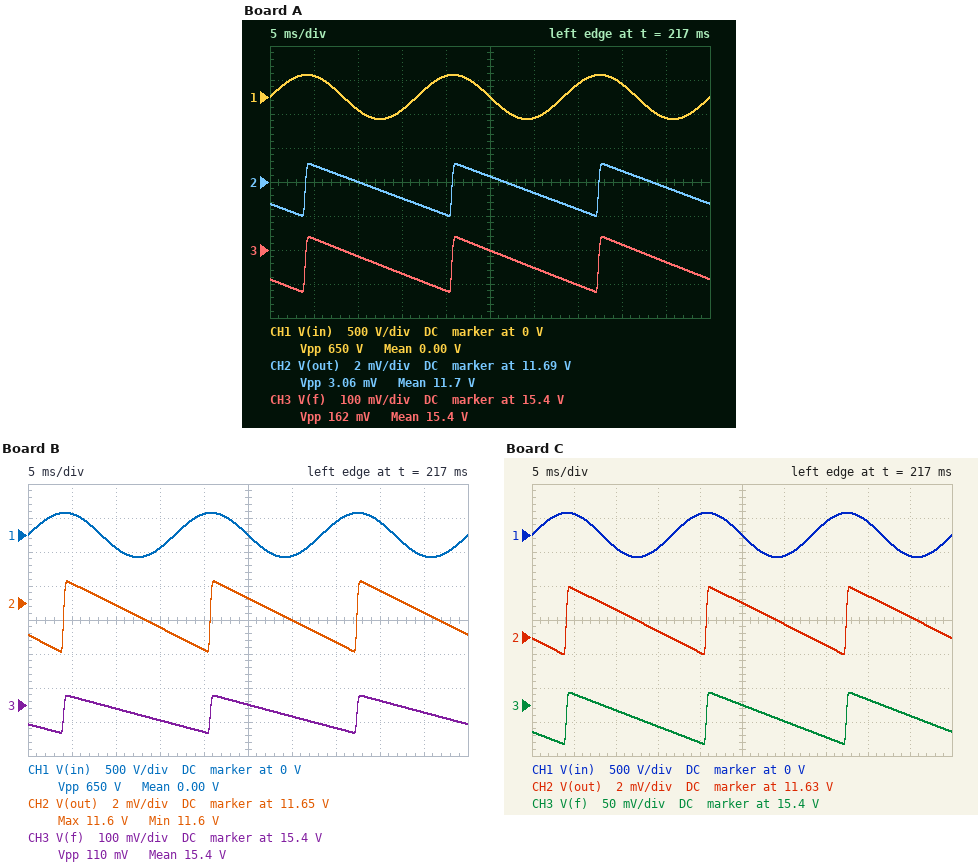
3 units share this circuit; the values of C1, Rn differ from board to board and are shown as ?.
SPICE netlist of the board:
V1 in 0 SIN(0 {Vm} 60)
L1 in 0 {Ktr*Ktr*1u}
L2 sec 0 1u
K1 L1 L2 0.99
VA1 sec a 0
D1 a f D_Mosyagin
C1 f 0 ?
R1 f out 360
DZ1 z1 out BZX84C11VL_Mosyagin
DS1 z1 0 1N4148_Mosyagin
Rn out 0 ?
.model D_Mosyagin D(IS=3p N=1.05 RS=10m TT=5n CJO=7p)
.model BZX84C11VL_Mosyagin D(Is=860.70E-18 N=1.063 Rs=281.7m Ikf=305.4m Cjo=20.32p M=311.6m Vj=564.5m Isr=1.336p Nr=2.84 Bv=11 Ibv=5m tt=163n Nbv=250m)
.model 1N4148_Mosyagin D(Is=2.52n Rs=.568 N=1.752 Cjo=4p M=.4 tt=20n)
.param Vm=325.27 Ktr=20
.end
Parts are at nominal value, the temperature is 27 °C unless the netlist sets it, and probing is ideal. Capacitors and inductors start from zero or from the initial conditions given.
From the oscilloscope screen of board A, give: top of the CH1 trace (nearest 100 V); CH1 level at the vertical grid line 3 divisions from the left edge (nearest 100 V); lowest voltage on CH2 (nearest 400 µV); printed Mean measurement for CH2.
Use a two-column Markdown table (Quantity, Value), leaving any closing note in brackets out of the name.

| Quantity | Value |
|---|---|
| top of the CH1 trace | 300 V |
| CH1 level at the vertical grid line 3 divisions from the left edge | -200 V |
| lowest voltage on CH2 | 11.6900 V |
| printed Mean measurement for CH2 | 11.7 V |
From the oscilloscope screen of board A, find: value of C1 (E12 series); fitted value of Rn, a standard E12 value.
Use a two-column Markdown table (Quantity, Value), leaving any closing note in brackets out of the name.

| Quantity | Value |
|---|---|
| value of C1 | 1 mF |
| fitted value of Rn, a standard E12 value | 6.8 kΩ |
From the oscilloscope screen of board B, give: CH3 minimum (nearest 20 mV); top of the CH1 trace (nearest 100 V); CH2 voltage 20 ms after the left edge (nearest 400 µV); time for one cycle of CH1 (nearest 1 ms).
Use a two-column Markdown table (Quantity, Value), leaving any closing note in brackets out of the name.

| Quantity | Value |
|---|---|
| CH3 minimum | 15.32 V |
| top of the CH1 trace | 300 V |
| CH2 voltage 20 ms after the left edge | 11.6452 V |
| time for one cycle of CH1 | 17 ms |
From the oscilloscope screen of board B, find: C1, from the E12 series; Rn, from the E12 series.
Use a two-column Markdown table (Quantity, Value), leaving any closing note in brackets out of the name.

| Quantity | Value |
|---|---|
| C1, from the E12 series | 1.5 mF |
| Rn, from the E12 series | 1.8 kΩ |
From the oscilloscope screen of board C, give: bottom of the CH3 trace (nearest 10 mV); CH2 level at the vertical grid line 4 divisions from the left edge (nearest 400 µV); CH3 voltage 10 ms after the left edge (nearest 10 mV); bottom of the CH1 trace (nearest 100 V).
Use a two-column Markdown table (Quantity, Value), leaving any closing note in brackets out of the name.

| Quantity | Value |
|---|---|
| bottom of the CH3 trace | 15.34 V |
| CH2 level at the vertical grid line 4 divisions from the left edge | 11.6252 V |
| CH3 voltage 10 ms after the left edge | 15.39 V |
| bottom of the CH1 trace | -300 V |
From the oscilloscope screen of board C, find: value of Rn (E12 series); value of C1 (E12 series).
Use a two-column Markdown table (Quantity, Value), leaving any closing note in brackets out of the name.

| Quantity | Value |
|---|---|
| value of Rn | 1.5 kΩ |
| value of C1 | 2.2 mF |
